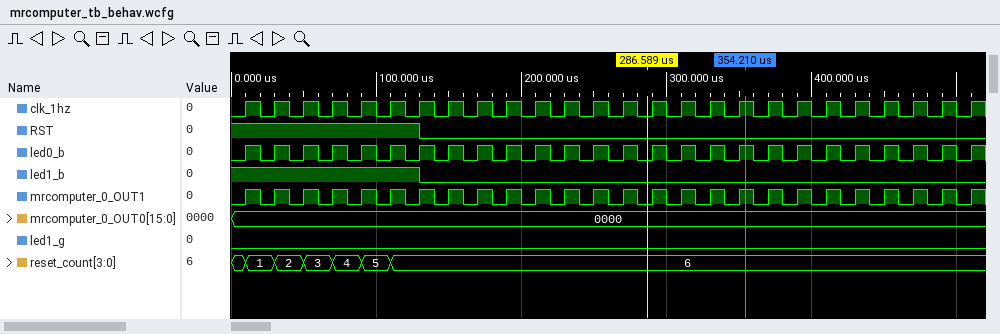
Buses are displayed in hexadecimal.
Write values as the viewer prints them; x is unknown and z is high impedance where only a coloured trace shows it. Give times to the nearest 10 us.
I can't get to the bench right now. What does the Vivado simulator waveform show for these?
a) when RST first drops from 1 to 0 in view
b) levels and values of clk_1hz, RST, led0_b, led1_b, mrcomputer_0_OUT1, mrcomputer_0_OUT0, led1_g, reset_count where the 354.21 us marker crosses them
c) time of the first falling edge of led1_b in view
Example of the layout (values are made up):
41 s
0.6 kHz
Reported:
130 us
clk_1hz=1, RST=0, led0_b=1, led1_b=0, mrcomputer_0_OUT1=1, mrcomputer_0_OUT0=0000, led1_g=0, reset_count=6
130 us
